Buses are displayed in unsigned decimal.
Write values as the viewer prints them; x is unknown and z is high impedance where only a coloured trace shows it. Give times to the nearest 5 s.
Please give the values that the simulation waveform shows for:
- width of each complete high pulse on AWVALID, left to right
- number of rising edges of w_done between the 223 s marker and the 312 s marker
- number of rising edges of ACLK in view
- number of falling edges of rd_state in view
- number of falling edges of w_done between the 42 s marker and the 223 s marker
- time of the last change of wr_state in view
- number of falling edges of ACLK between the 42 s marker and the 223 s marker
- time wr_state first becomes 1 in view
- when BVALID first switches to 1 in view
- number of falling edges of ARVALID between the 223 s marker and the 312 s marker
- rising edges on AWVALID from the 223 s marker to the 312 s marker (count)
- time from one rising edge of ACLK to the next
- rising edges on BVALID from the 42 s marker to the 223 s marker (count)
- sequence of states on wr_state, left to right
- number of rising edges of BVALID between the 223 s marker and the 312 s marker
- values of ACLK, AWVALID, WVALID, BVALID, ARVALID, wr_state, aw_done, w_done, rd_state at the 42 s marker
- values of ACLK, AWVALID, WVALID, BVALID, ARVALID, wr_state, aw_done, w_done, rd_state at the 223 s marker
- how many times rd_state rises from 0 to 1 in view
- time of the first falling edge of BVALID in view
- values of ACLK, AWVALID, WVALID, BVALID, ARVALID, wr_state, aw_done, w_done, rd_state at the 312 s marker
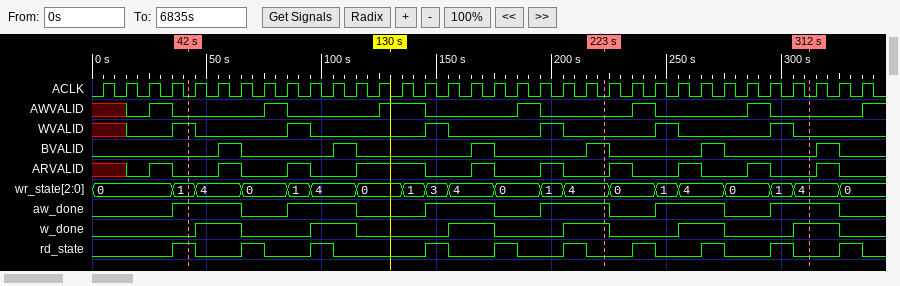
10 s, 10 s, 20 s, 10 s, 10 s, 10 s
2
34
10
3
325 s
18
35 s
55 s
3
2
10 s
4
0, 1, 4, 0, 1, 4, 0, 1, 3, 4, 0, 1, 4, 0, 1, 4, 0, 1, 4, 0
1
ACLK=0, AWVALID=0, WVALID=1, BVALID=0, ARVALID=0, wr_state=1, aw_done=1, w_done=0, rd_state=1
ACLK=0, AWVALID=0, WVALID=0, BVALID=1, ARVALID=0, wr_state=4, aw_done=1, w_done=1, rd_state=0
10
65 s
ACLK=0, AWVALID=0, WVALID=0, BVALID=0, ARVALID=0, wr_state=4, aw_done=1, w_done=1, rd_state=0
